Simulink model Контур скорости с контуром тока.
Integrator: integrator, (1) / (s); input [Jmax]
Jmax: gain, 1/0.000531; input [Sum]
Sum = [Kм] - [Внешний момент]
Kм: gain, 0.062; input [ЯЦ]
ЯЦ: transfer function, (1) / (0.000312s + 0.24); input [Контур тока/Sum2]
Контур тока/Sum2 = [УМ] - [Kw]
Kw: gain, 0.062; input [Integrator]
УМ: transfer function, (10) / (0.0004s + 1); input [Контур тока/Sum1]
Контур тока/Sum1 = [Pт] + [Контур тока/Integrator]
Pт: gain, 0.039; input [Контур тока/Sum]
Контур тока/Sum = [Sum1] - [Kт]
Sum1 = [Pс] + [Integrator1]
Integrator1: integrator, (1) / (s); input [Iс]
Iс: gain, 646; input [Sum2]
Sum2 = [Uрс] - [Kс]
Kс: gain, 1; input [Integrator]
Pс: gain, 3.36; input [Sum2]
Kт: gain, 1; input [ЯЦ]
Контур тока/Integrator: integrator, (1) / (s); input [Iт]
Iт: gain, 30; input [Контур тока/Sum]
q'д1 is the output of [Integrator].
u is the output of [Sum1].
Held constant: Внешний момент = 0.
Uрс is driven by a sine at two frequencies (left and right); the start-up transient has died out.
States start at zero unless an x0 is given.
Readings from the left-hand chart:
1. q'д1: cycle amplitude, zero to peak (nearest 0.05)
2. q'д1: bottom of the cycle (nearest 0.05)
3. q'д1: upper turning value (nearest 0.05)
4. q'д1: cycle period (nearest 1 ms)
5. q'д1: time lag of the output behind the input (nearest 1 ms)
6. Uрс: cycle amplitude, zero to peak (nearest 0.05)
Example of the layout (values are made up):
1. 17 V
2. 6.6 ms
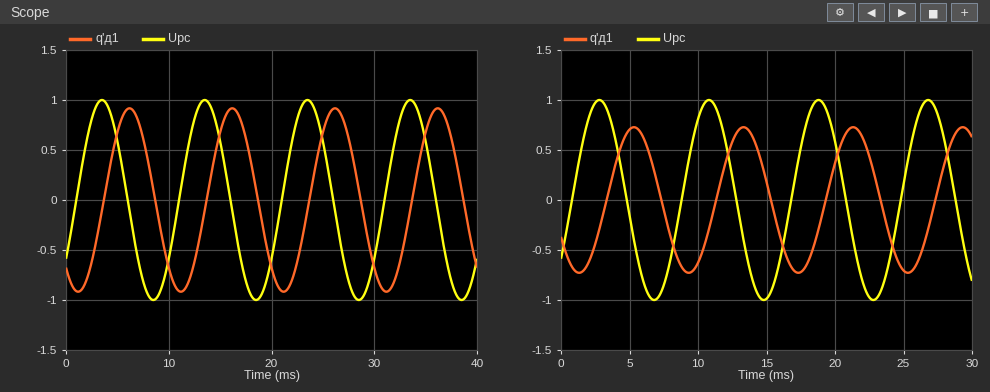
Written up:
1. 0.90
2. -0.90
3. 0.90
4. 10 ms
5. 3 ms
6. 1.00
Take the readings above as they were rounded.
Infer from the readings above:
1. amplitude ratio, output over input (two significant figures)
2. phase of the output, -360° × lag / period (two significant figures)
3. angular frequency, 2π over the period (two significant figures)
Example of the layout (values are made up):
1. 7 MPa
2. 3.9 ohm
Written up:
1. 0.90
2. -110°
3. 0.63 rad/ms
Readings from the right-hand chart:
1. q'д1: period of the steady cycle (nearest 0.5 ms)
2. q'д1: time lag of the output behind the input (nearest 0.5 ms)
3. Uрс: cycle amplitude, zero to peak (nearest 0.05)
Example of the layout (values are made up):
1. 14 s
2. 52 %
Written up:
1. 8.0 ms
2. 2.5 ms
3. 1.00
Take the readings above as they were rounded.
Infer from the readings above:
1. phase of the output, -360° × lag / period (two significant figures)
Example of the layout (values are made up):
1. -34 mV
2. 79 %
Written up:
1. -110°
